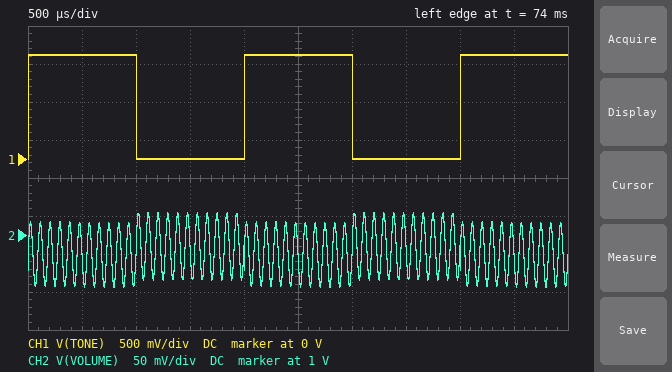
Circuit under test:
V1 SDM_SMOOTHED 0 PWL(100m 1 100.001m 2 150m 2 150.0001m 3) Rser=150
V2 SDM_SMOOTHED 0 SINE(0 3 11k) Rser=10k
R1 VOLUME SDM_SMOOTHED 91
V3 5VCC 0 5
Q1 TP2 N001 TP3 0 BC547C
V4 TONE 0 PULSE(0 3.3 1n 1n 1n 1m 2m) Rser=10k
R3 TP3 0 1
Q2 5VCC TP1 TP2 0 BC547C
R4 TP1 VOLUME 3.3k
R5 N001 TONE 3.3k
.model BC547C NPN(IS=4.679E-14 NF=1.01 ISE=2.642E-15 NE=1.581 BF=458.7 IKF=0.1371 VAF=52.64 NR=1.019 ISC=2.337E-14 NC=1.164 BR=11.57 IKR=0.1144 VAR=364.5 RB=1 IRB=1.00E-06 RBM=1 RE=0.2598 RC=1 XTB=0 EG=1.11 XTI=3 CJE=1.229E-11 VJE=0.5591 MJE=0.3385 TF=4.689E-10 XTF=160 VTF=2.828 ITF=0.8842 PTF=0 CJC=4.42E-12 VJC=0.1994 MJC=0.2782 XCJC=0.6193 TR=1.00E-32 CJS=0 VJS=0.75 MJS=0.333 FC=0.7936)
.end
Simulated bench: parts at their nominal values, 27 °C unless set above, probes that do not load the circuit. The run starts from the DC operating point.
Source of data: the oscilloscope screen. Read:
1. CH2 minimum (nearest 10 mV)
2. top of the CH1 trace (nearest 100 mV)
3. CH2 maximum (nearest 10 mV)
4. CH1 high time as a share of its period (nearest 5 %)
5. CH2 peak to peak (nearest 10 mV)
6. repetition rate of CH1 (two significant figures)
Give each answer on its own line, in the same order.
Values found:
930 mV
1.4 V
1.03 V
50 %
100 mV
500 Hz
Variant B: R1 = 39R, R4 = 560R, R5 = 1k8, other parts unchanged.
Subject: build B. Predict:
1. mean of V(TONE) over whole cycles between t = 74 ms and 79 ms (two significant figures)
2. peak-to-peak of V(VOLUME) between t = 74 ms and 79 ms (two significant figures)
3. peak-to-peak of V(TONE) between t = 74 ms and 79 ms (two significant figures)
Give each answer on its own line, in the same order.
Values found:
580 mV
100 mV
1.2 V
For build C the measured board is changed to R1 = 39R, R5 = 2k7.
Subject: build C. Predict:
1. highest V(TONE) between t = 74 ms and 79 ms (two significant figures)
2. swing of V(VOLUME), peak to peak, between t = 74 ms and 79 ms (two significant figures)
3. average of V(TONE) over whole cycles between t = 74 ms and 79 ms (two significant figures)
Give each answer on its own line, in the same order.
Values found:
1.3 V
96 mV
640 mV
